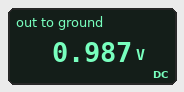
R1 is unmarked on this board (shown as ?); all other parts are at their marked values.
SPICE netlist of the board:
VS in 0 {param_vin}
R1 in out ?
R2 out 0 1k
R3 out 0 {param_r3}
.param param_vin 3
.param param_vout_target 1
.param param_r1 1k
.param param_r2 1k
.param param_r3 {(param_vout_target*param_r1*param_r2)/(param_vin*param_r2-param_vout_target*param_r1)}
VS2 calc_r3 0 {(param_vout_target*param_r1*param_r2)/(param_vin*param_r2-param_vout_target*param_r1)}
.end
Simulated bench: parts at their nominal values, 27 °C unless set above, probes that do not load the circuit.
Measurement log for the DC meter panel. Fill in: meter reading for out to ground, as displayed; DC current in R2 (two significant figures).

0.987 V
990 µA
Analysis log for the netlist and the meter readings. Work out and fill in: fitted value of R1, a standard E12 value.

680 Ω
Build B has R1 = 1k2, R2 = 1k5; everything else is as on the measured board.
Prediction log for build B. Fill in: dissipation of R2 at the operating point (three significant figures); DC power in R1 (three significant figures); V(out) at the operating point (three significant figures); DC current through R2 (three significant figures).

340 µW
4.35 mW
714 mV
476 µA
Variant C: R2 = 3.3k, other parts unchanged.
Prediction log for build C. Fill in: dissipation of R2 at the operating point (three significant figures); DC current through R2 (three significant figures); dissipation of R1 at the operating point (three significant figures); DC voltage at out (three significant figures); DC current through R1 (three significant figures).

414 µW
354 µA
4.93 mW
1.17 V
2.69 mA
